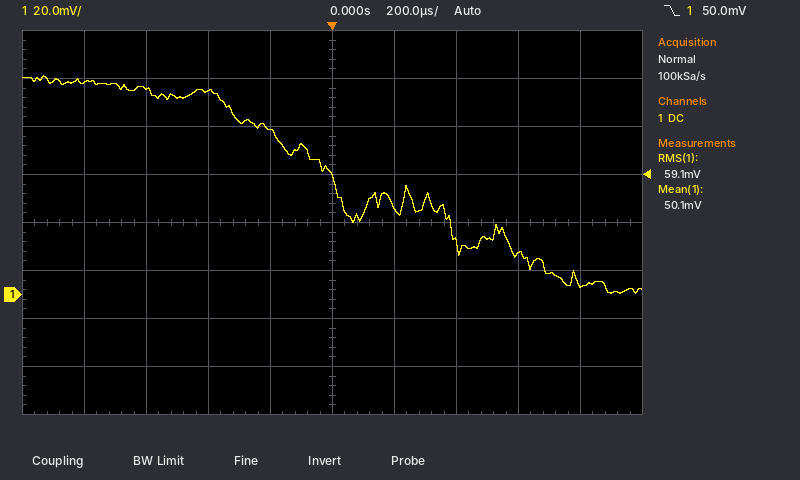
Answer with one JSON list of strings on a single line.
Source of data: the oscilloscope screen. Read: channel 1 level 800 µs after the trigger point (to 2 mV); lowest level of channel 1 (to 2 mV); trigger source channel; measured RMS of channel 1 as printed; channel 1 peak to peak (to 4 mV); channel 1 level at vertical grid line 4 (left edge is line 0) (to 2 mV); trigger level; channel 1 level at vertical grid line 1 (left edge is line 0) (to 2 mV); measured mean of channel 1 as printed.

["4 mV", "0 mV", "channel 1", "59.1 mV", "92 mV", "68 mV", "50.0 mV", "88 mV", "50.1 mV"]
